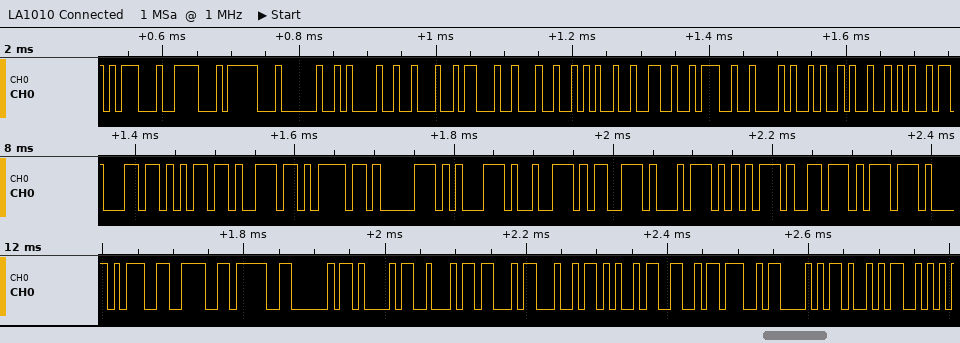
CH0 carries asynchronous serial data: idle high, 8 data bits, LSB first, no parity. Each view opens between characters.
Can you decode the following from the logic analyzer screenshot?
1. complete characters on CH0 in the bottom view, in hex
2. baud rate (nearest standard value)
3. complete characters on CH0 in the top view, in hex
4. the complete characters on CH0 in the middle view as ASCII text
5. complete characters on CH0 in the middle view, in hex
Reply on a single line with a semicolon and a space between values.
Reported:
9D, 9E, 9F, A0, A1, A2, A3, A4, A5, A6, A7, A8, A9; 115200 baud; 1D, 1E, 1F, 20, 21, 22, 23, 24, 25, 26, 27, 28, 29, 2A; "lmnopqrstuvw"; 6C, 6D, 6E, 6F, 70, 71, 72, 73, 74, 75, 76, 77
